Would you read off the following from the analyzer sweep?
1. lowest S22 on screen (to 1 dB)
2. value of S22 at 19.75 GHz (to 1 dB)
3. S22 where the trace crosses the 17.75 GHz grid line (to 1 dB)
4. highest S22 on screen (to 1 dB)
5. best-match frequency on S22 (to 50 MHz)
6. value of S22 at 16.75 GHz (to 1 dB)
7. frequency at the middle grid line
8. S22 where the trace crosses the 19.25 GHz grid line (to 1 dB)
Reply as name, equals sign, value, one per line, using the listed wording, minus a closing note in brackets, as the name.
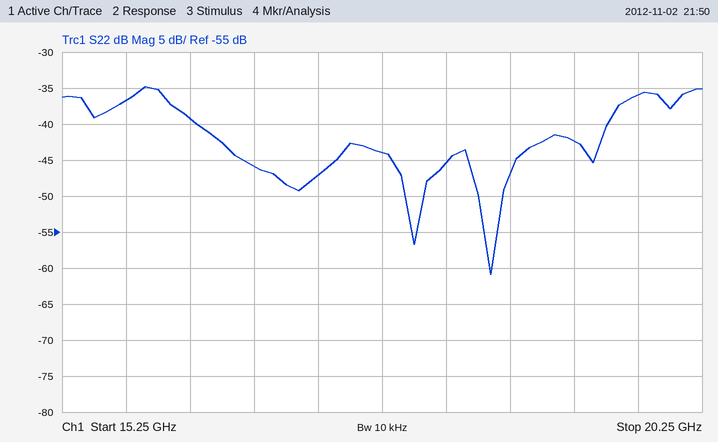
lowest S22 on screen = -61 dB
value of S22 at 19.75 GHz = -36 dB
S22 where the trace crosses the 17.75 GHz grid line = -44 dB
highest S22 on screen = -35 dB
best-match frequency on S22 = 18.60 GHz
value of S22 at 16.75 GHz = -46 dB
frequency at the middle grid line = 17.75 GHz
S22 where the trace crosses the 19.25 GHz grid line = -42 dB
